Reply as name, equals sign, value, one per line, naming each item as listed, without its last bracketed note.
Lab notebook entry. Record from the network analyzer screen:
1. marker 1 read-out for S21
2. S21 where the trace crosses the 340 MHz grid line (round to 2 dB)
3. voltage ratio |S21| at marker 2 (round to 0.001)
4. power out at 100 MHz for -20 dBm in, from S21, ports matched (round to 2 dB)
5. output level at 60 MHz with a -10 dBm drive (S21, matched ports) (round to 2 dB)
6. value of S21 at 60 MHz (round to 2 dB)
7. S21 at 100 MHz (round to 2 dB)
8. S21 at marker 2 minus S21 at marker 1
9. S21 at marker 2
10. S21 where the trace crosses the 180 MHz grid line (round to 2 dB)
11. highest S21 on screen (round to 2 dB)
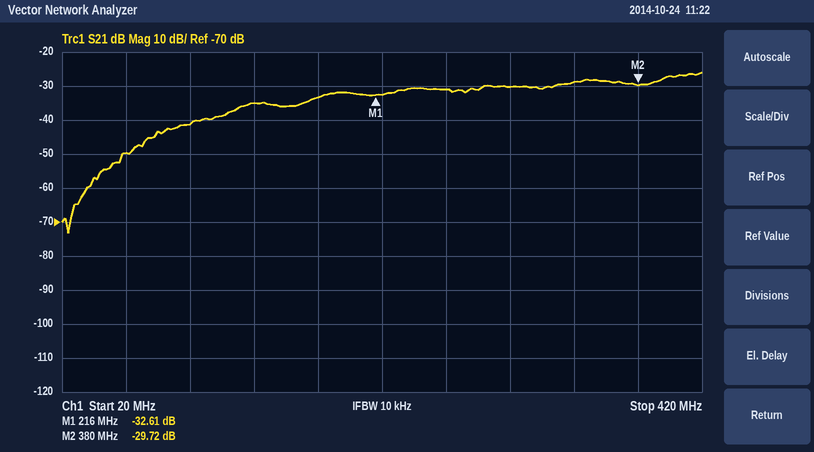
marker 1 read-out for S21 = -32.61 dB
S21 where the trace crosses the 340 MHz grid line = -28 dB
voltage ratio |S21| at marker 2 = 0.033
power out at 100 MHz for -20 dBm in, from S21, ports matched = -62 dBm
output level at 60 MHz with a -10 dBm drive (S21, matched ports) = -60 dBm
value of S21 at 60 MHz = -50 dB
S21 at 100 MHz = -42 dB
S21 at marker 2 minus S21 at marker 1 = 2.89 dB
S21 at marker 2 = -29.72 dB
S21 where the trace crosses the 180 MHz grid line = -34 dB
highest S21 on screen = -26 dB
